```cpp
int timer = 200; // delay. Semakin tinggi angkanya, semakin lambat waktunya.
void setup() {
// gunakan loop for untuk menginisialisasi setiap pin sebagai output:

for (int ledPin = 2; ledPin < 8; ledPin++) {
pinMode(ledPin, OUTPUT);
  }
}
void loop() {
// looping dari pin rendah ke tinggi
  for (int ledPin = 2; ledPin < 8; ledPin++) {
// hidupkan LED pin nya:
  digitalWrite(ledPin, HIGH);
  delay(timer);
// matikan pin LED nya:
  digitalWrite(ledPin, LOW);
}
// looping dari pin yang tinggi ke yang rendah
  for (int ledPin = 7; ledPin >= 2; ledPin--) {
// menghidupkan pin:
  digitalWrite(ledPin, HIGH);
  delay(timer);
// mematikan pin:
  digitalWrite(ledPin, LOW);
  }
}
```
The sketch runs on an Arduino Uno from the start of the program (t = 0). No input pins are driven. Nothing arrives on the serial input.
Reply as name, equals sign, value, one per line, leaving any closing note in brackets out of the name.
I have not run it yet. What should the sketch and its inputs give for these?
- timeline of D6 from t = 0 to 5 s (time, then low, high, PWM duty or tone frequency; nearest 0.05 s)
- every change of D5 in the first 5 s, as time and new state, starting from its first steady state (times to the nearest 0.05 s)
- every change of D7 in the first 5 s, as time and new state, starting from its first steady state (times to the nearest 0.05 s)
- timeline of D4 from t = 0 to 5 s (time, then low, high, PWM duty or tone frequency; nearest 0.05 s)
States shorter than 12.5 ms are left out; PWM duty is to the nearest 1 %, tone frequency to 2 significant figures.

timeline of D6 from t = 0 to 5 s = 0 s low; 0.8 s high; 1 s low; 1.4 s high; 1.6 s low; 3.2 s high; 3.4 s low; 3.8 s high; 4 s low
every change of D5 in the first 5 s, as time and new state, starting from its first steady state = 0 s low; 0.6 s high; 0.8 s low; 1.6 s high; 1.8 s low; 3 s high; 3.2 s low; 4 s high; 4.2 s low
every change of D7 in the first 5 s, as time and new state, starting from its first steady state = 0 s low; 1 s high; 1.4 s low; 3.4 s high; 3.8 s low
timeline of D4 from t = 0 to 5 s = 0 s low; 0.4 s high; 0.6 s low; 1.8 s high; 2 s low; 2.8 s high; 3 s low; 4.2 s high; 4.4 s low
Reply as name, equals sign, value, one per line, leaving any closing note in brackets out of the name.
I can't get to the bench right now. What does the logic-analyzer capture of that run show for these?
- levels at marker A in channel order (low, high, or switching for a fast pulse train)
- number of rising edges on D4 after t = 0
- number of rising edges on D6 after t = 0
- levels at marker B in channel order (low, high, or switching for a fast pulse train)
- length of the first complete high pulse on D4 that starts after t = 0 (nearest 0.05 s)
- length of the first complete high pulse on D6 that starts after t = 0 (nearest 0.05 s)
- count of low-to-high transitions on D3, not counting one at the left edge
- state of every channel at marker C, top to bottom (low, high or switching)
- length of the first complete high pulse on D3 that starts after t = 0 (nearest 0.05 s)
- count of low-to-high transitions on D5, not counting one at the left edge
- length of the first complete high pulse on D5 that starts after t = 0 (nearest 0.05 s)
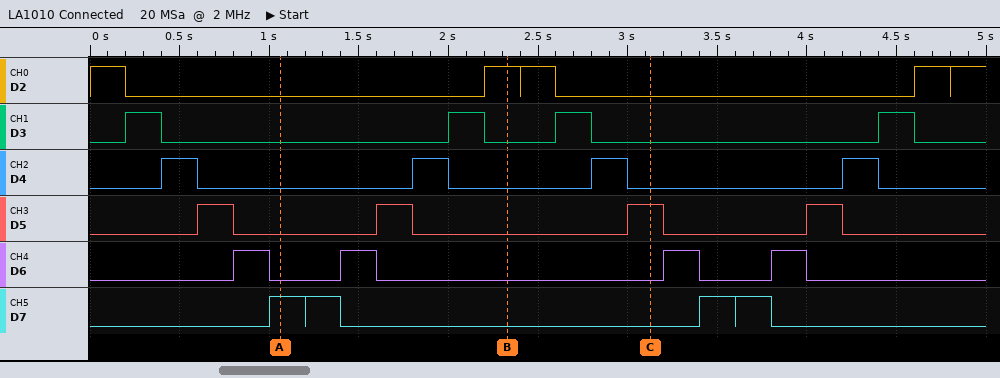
levels at marker A in channel order = D2 low, D3 low, D4 low, D5 low, D6 low, D7 high
number of rising edges on D4 after t = 0 = 4
number of rising edges on D6 after t = 0 = 4
levels at marker B in channel order = D2 high, D3 low, D4 low, D5 low, D6 low, D7 low
length of the first complete high pulse on D4 that starts after t = 0 = 0.20 s
length of the first complete high pulse on D6 that starts after t = 0 = 0.20 s
count of low-to-high transitions on D3, not counting one at the left edge = 4
state of every channel at marker C, top to bottom = D2 low, D3 low, D4 low, D5 high, D6 low, D7 low
length of the first complete high pulse on D3 that starts after t = 0 = 0.20 s
count of low-to-high transitions on D5, not counting one at the left edge = 4
length of the first complete high pulse on D5 that starts after t = 0 = 0.20 s
